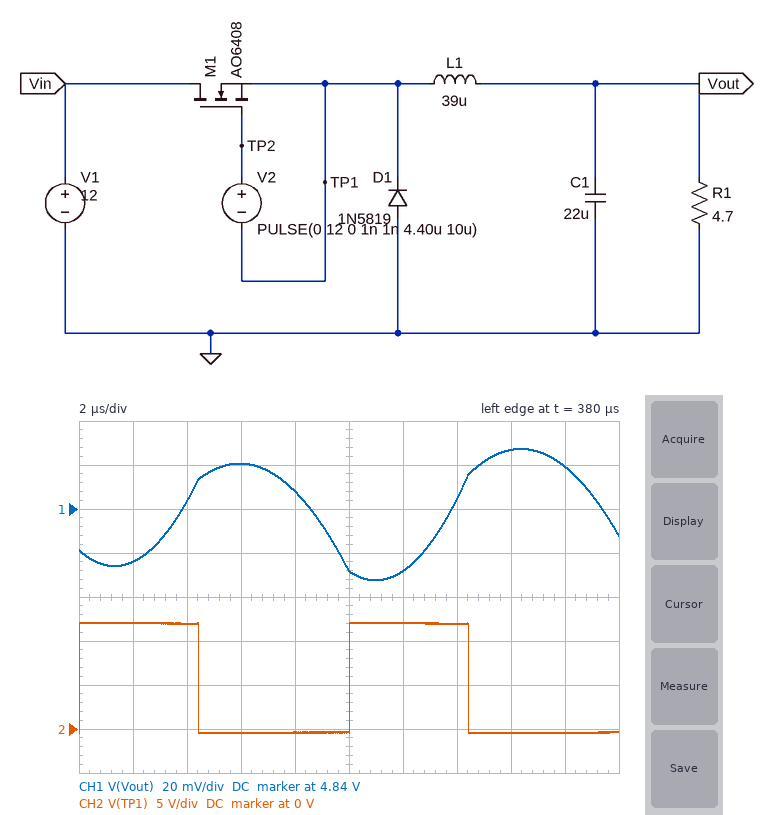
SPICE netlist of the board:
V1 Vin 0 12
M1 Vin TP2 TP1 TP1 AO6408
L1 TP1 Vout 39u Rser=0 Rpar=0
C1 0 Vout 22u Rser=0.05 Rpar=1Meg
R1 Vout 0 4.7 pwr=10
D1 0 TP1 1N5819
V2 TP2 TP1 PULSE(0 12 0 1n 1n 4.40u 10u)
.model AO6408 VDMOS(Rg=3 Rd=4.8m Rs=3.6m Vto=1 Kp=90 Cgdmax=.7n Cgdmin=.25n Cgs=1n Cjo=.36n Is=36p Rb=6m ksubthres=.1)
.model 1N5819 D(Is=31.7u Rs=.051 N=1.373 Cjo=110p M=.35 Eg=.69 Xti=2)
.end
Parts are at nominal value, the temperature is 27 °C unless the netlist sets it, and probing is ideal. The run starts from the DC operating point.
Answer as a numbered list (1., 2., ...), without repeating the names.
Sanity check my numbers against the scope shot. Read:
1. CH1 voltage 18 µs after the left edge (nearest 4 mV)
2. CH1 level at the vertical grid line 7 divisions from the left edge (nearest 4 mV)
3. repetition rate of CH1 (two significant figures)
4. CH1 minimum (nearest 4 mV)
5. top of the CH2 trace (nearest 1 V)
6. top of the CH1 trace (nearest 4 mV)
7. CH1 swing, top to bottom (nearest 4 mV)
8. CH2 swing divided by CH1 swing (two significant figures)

1. 4.860 V
2. 4.844 V
3. 100 kHz
4. 4.808 V
5. 12 V
6. 4.868 V
7. 60 mV
8. 210
